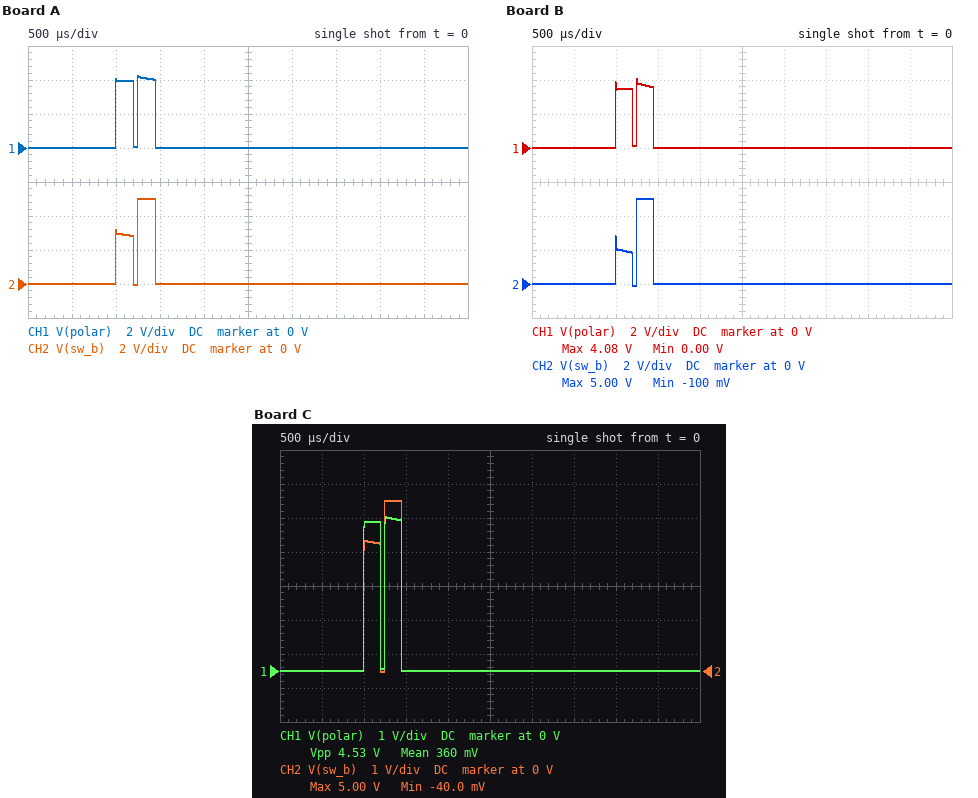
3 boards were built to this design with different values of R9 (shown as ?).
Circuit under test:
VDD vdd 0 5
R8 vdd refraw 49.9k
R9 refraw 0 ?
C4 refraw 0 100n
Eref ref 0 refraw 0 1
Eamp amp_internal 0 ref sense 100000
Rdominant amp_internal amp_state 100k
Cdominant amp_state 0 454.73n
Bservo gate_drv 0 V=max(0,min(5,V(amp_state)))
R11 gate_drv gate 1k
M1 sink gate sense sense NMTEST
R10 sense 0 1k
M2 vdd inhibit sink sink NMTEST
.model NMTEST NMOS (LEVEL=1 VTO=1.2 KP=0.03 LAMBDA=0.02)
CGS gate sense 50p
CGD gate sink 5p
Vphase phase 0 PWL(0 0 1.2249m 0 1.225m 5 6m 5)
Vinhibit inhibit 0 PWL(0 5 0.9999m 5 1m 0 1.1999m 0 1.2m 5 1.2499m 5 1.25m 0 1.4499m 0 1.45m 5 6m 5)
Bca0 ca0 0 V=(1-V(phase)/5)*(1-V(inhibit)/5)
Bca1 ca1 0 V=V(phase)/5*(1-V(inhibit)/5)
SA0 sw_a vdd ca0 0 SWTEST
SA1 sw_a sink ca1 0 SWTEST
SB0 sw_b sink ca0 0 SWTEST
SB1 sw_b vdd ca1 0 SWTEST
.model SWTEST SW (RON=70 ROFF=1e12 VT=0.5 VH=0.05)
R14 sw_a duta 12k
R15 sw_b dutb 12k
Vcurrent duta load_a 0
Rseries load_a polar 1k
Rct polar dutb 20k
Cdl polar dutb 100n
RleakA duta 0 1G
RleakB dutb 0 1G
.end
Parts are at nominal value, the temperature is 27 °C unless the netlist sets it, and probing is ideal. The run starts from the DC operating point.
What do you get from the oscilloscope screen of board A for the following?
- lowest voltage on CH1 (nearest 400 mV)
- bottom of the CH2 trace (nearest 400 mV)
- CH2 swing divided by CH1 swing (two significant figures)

0 V
0 V
1.2
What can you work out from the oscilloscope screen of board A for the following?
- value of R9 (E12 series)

820 Ω
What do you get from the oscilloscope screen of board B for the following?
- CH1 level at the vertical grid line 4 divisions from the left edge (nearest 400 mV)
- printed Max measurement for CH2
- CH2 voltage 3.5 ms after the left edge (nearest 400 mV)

0 V
5.00 V
0 V
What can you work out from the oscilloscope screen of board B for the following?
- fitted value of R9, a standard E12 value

1.2 kΩ
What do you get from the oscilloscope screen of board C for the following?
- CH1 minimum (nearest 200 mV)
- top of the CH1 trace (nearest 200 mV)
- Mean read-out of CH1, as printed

0 V
4.6 V
360 mV
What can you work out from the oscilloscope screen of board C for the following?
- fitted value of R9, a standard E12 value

470 Ω
